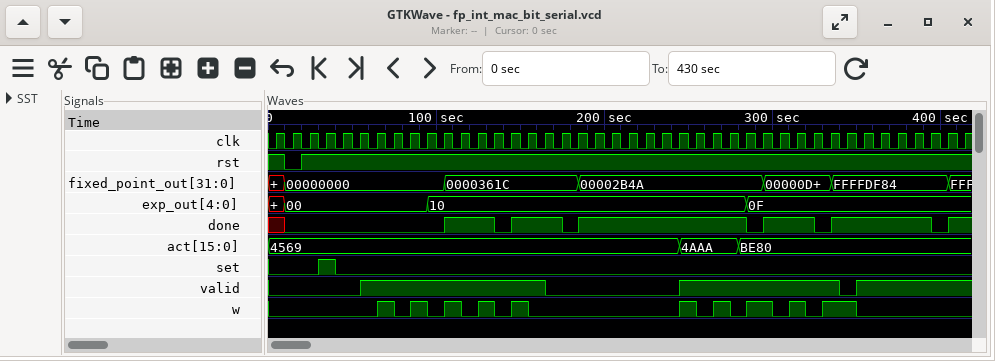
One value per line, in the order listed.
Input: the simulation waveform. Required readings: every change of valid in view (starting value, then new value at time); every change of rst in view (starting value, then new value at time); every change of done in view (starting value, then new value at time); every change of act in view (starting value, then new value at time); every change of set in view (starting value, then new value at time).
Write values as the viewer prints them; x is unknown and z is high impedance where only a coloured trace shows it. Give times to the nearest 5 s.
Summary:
0, 1 at 55 s, 0 at 165 s, 1 at 245 s, 0 at 340 s, 1 at 350 s
1, 0 at 10 s, 1 at 20 s
x, 0 at 10 s, 1 at 105 s, 0 at 135 s, 1 at 145 s, 0 at 175 s, 1 at 185 s, 0 at 285 s, 1 at 295 s, 0 at 325 s, 1 at 335 s, 0 at 395 s, 1 at 405 s
4569, 4AAA at 245 s, BE80 at 280 s
0, 1 at 30 s, 0 at 40 s
